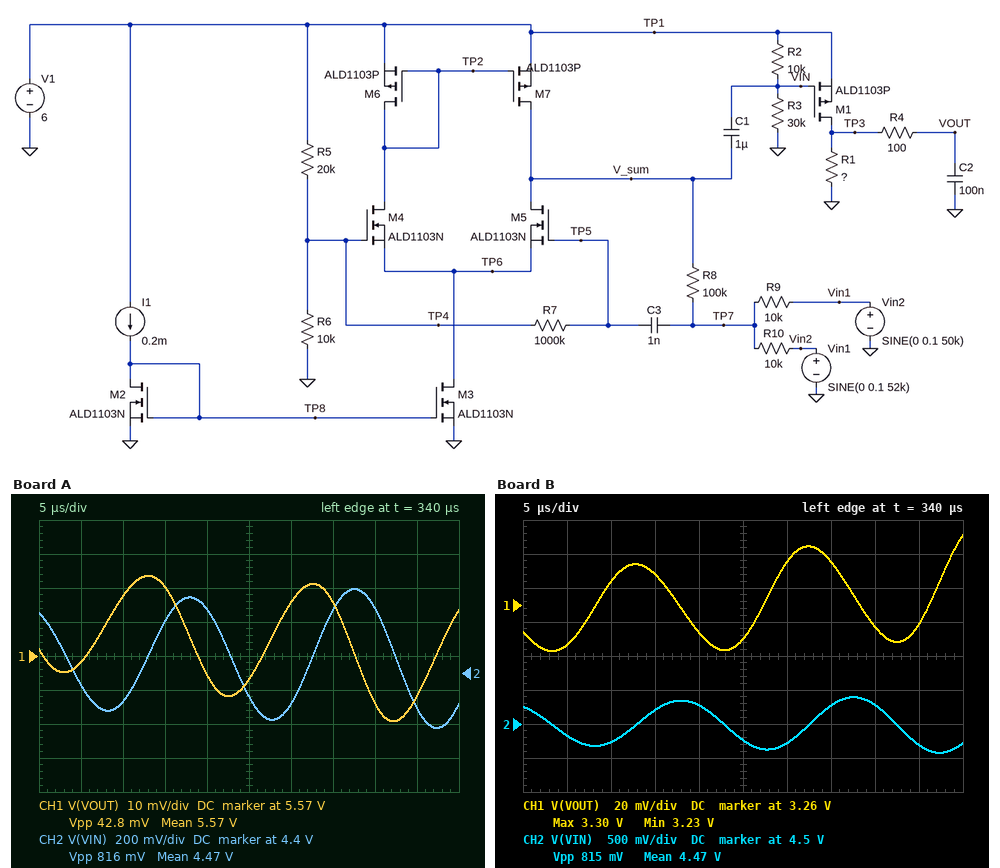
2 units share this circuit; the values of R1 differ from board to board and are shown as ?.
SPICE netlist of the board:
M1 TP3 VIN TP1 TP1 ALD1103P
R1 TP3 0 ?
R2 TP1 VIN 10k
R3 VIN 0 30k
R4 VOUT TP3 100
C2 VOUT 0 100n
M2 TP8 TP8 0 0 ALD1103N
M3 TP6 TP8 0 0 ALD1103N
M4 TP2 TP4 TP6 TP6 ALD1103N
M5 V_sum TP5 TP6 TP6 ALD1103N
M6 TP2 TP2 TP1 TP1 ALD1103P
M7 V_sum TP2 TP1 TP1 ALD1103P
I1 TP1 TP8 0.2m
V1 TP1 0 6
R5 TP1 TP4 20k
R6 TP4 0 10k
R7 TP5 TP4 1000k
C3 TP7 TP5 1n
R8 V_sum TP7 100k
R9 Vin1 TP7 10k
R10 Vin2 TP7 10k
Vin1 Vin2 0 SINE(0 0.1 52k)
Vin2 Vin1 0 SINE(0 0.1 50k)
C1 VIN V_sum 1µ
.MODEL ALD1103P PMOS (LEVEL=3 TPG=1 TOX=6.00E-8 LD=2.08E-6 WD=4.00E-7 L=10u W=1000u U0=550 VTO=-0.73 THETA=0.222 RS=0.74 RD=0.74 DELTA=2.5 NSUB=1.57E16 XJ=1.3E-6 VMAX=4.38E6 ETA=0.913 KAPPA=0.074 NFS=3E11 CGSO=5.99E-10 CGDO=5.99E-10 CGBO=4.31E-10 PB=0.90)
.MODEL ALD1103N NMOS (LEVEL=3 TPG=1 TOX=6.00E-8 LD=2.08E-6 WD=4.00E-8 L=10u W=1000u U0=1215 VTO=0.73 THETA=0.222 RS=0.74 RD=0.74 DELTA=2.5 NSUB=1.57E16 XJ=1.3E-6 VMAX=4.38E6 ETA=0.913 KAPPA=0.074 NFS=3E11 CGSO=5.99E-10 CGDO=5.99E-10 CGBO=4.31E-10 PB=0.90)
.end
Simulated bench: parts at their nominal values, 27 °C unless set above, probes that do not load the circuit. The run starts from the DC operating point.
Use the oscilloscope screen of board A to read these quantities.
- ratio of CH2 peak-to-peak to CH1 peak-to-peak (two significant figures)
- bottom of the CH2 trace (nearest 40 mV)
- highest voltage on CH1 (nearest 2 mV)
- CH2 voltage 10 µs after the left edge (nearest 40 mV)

19
4.08 V
5.594 V
4.24 V
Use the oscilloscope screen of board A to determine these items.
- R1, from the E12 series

5.6 kΩ
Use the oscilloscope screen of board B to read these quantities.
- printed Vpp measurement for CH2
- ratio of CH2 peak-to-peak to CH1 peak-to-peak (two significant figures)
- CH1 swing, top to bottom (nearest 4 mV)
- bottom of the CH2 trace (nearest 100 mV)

815 mV
12
68 mV
4.1 V
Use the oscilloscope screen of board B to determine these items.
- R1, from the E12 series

2.7 kΩ
